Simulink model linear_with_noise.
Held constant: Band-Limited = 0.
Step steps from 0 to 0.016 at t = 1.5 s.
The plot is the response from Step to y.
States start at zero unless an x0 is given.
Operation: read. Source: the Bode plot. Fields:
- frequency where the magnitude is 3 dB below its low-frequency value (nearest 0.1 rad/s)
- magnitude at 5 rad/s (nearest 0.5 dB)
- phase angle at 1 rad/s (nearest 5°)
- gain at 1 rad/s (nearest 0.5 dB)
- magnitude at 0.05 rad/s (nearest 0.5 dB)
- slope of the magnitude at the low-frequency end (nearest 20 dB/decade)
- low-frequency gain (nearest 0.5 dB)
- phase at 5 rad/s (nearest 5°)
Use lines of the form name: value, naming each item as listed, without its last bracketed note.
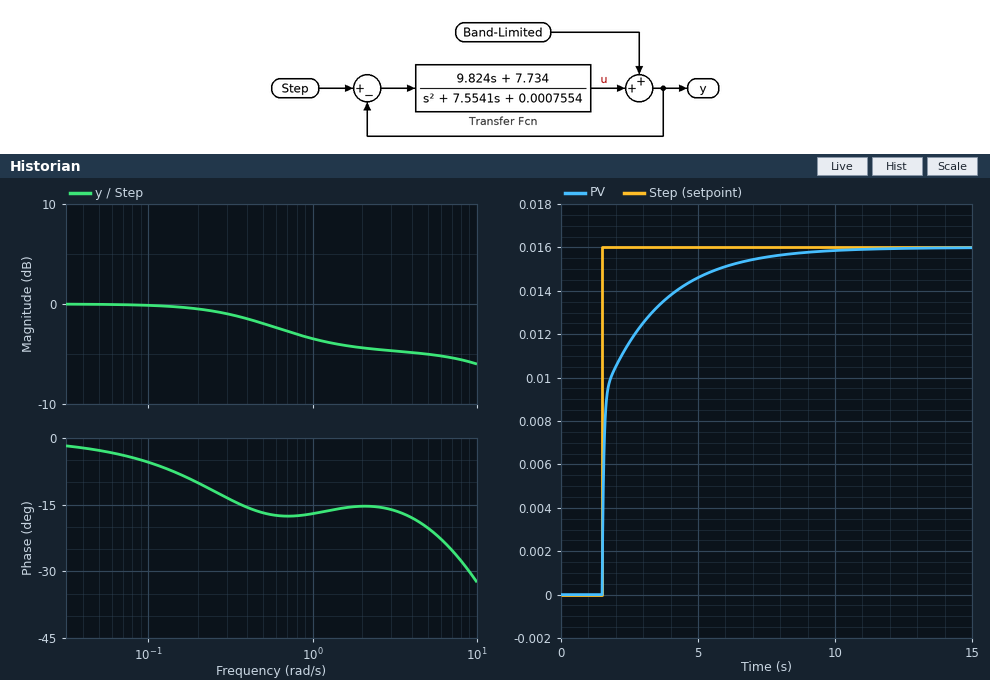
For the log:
frequency where the magnitude is 3 dB below its low-frequency value: 0.8 rad/s
magnitude at 5 rad/s: -5.0 dB
phase angle at 1 rad/s: -15°
gain at 1 rad/s: -3.5 dB
magnitude at 0.05 rad/s: 0.0 dB
slope of the magnitude at the low-frequency end: 0 dB/decade
low-frequency gain: 0.0 dB
phase at 5 rad/s: -20°
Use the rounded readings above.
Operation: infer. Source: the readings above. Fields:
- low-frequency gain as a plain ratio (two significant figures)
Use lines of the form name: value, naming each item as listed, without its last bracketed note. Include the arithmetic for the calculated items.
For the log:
low-frequency gain as a plain ratio: 10^(0 / 20) = 1.0
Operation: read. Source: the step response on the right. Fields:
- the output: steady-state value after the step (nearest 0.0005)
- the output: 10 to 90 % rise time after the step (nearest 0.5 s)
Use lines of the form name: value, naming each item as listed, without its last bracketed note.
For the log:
the output: steady-state value after the step: 0.0160
the output: 10 to 90 % rise time after the step: 3.0 s
